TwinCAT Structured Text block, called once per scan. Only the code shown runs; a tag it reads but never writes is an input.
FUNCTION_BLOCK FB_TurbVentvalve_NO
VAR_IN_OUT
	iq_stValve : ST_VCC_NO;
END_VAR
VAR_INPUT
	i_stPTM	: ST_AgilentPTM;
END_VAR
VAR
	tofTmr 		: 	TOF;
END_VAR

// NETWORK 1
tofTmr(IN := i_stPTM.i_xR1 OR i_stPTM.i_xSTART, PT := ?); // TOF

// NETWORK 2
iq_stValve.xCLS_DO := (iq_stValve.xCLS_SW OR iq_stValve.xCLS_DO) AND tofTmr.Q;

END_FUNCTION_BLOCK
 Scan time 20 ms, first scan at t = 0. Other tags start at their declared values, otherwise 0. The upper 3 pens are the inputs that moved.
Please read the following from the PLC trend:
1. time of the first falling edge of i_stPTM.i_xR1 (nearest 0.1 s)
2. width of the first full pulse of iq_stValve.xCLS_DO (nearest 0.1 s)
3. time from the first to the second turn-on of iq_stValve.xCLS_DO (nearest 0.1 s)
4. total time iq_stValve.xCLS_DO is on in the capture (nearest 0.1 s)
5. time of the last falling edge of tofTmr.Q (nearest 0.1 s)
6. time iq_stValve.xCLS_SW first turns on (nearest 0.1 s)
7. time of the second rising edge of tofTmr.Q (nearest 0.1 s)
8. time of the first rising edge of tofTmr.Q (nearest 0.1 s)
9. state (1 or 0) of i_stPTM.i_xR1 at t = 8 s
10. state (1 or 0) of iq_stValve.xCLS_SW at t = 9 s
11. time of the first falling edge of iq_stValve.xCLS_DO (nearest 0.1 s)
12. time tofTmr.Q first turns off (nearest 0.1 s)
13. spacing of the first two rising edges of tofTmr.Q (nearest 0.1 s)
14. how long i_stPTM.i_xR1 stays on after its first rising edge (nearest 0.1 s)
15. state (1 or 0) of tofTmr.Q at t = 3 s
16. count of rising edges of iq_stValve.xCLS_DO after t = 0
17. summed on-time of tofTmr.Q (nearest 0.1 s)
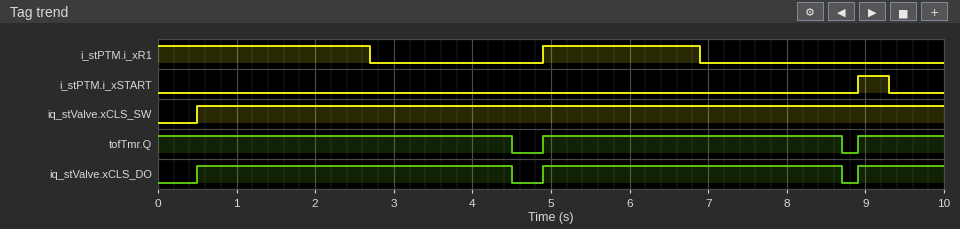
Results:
2.7 s
4.0 s
4.4 s
8.9 s
8.7 s
0.5 s
8.9 s
4.9 s
0
1
4.5 s
4.5 s
4.0 s
2.0 s
1
3
9.4 s
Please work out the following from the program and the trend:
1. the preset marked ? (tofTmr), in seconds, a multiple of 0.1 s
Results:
1.8 s
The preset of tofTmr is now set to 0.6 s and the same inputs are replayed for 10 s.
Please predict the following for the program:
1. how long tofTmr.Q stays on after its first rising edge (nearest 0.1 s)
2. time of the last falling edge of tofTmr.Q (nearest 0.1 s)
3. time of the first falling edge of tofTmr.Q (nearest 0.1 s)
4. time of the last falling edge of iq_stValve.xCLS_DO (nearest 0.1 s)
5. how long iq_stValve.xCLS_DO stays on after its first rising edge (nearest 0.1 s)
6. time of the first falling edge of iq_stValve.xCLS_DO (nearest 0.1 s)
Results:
2.6 s
9.9 s
3.3 s
9.9 s
2.8 s
3.3 s
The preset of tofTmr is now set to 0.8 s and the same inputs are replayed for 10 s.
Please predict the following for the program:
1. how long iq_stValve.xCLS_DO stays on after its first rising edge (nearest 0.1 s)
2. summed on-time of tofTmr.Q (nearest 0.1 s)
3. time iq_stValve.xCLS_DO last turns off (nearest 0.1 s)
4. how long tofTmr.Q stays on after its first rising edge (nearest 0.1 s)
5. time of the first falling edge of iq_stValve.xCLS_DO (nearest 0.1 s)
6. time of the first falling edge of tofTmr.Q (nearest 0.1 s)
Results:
3.0 s
7.4 s
7.7 s
2.8 s
3.5 s
3.5 s
